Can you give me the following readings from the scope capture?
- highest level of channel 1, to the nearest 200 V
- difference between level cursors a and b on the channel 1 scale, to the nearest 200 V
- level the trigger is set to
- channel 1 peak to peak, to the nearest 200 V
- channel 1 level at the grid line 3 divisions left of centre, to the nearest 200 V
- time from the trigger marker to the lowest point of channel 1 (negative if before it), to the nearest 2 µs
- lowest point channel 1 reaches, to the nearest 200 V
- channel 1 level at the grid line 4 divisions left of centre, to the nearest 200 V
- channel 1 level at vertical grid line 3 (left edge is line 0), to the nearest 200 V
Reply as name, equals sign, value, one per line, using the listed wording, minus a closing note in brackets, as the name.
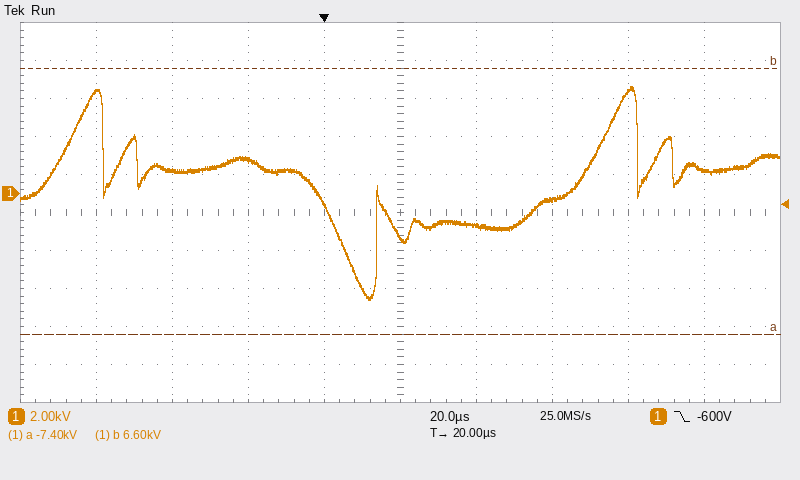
highest level of channel 1, to the nearest 200 V = 5.6 kV
difference between level cursors a and b on the channel 1 scale, to the nearest 200 V = 14.0 kV
level the trigger is set to = -600 V
channel 1 peak to peak, to the nearest 200 V = 11.2 kV
channel 1 level at the grid line 3 divisions left of centre, to the nearest 200 V = 1.2 kV
time from the trigger marker to the lowest point of channel 1 (negative if before it), to the nearest 2 µs = +12 µs
lowest point channel 1 reaches, to the nearest 200 V = -5.6 kV
channel 1 level at the grid line 4 divisions left of centre, to the nearest 200 V = 5.4 kV
channel 1 level at vertical grid line 3 (left edge is line 0), to the nearest 200 V = 1.8 kV
